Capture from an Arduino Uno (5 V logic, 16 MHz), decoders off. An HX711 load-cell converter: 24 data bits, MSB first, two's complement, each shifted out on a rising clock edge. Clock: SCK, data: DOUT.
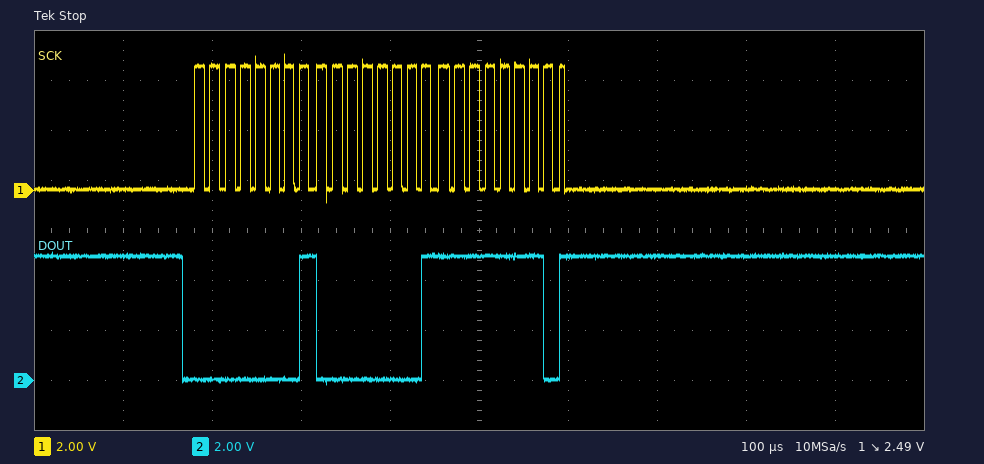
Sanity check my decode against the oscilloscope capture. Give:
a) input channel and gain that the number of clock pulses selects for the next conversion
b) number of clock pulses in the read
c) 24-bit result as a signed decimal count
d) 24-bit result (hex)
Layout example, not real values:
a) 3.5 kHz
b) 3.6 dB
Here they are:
a) channel A, gain 128
b) 25
c) 66046
d) 0x0101FE
